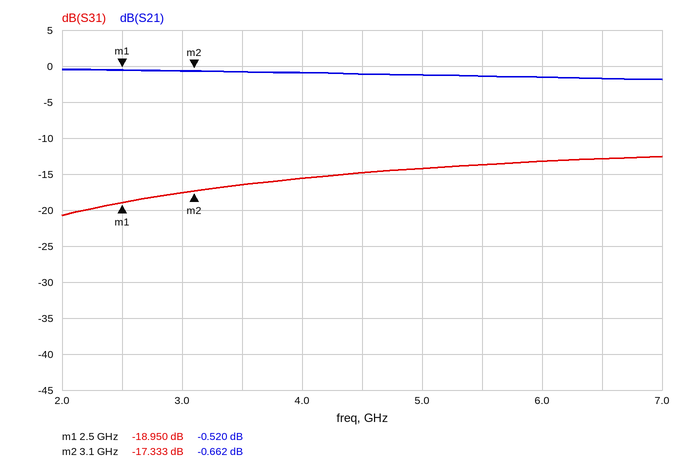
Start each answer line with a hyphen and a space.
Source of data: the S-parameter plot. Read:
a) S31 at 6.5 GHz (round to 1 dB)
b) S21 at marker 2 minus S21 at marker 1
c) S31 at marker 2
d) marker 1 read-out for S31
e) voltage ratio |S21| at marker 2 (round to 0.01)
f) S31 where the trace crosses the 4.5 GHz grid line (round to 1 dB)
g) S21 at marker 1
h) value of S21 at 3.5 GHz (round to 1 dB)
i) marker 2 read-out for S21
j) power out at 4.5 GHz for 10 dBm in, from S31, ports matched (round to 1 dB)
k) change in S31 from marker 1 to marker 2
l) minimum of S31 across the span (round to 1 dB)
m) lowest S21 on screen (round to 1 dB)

- -13 dB
- -0.142 dB
- -17.333 dB
- -18.950 dB
- 0.93
- -15 dB
- -0.520 dB
- -1 dB
- -0.662 dB
- -5 dBm
- 1.617 dB
- -21 dB
- -2 dB
